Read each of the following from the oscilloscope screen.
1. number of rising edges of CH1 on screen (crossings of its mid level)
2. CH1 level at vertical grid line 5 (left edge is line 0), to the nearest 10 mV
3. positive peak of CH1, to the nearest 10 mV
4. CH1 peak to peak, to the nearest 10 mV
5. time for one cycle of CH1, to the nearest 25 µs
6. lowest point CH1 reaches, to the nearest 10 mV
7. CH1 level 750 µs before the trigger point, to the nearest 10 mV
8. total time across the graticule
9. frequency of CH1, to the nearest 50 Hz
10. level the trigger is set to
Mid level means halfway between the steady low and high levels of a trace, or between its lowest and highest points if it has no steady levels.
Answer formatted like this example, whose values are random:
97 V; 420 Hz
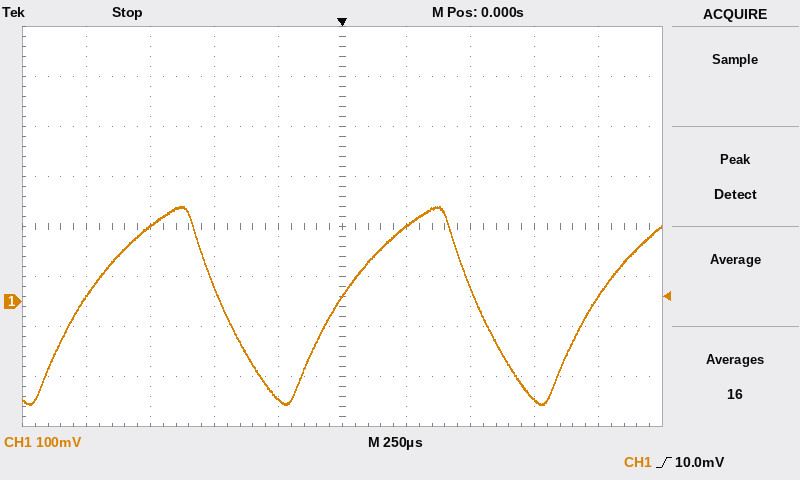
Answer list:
3; 10 mV; 190 mV; 400 mV; 1.000 ms; -210 mV; 150 mV; 2.5 ms; 1.00 kHz; 10.0 mV
